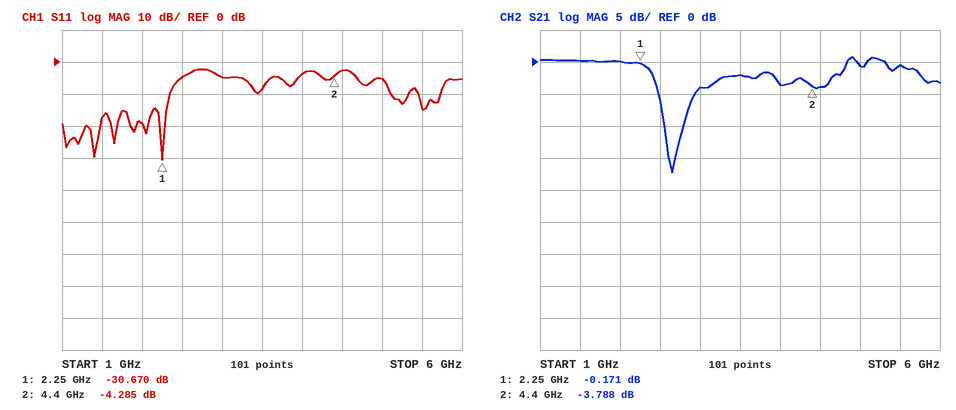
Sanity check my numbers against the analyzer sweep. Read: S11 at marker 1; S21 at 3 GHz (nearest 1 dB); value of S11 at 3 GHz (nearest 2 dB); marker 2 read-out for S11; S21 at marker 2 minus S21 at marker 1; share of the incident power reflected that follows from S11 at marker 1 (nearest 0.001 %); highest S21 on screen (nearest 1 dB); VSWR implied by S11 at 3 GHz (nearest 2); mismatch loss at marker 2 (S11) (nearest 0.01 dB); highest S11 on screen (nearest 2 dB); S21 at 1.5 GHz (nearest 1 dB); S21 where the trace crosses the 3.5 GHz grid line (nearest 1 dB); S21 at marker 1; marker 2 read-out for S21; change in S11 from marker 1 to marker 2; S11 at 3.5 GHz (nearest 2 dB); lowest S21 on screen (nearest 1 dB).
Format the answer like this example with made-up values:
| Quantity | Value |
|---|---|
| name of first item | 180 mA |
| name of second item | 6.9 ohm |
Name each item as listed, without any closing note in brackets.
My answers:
| Quantity | Value |
|---|---|
| S11 at marker 1 | -30.670 dB |
| S21 at 3 GHz | -4 dB |
| value of S11 at 3 GHz | -4 dB |
| marker 2 read-out for S11 | -4.285 dB |
| S21 at marker 2 minus S21 at marker 1 | -3.617 dB |
| share of the incident power reflected that follows from S11 at marker 1 | 0.086 % |
| highest S21 on screen | 1 dB |
| VSWR implied by S11 at 3 GHz | 4 |
| mismatch loss at marker 2 (S11) | 2.03 dB |
| highest S11 on screen | -2 dB |
| S21 at 1.5 GHz | 0 dB |
| S21 where the trace crosses the 3.5 GHz grid line | -2 dB |
| S21 at marker 1 | -0.171 dB |
| marker 2 read-out for S21 | -3.788 dB |
| change in S11 from marker 1 to marker 2 | 26.385 dB |
| S11 at 3.5 GHz | -8 dB |
| lowest S21 on screen | -17 dB |
